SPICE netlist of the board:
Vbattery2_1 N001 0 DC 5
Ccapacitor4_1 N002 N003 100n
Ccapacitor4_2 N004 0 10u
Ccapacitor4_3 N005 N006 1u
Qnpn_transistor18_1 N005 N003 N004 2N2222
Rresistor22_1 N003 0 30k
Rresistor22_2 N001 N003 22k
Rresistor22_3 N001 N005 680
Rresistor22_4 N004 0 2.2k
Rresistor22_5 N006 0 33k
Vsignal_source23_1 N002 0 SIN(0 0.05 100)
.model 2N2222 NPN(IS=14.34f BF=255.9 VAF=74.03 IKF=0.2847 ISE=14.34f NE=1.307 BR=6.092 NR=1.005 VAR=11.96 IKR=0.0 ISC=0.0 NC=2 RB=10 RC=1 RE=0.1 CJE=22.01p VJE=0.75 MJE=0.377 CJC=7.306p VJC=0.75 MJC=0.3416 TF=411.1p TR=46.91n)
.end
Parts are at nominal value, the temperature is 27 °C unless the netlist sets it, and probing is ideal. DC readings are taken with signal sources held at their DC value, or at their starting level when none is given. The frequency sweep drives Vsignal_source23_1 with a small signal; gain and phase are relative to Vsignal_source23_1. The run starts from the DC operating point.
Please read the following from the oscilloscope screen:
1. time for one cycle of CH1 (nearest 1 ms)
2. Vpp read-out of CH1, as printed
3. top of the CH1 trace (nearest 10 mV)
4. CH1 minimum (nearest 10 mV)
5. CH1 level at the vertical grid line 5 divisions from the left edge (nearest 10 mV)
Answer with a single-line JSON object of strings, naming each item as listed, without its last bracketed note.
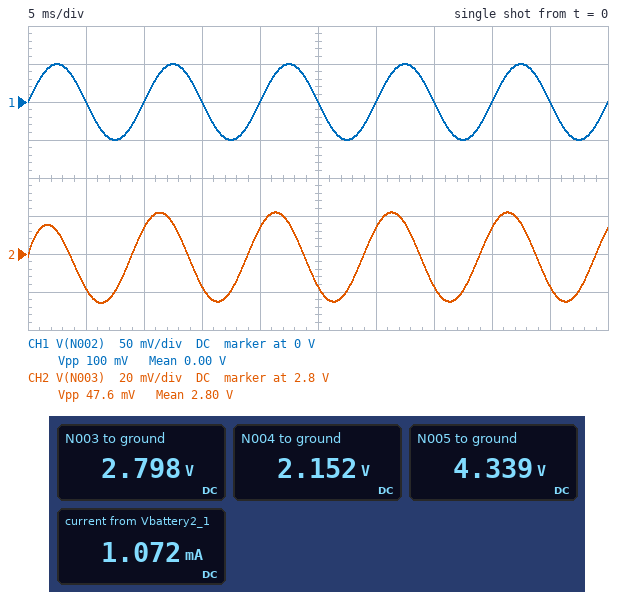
{"time for one cycle of CH1": "10 ms", "Vpp read-out of CH1, as printed": "100 mV", "top of the CH1 trace": "50 mV", "CH1 minimum": "-50 mV", "CH1 level at the vertical grid line 5 divisions from the left edge": "0 V"}
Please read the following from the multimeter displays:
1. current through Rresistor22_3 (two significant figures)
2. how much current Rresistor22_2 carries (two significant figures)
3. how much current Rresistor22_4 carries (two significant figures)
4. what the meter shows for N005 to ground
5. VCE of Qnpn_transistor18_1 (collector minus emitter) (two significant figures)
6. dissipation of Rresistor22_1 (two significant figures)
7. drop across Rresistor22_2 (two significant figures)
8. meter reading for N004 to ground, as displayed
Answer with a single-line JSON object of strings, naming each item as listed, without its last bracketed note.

{"current through Rresistor22_3": "970 µA", "how much current Rresistor22_2 carries": "100 µA", "how much current Rresistor22_4 carries": "980 µA", "what the meter shows for N005 to ground": "4.339 V", "VCE of Qnpn_transistor18_1 (collector minus emitter)": "2.2 V", "dissipation of Rresistor22_1": "260 µW", "drop across Rresistor22_2": "2.2 V", "meter reading for N004 to ground, as displayed": "2.152 V"}
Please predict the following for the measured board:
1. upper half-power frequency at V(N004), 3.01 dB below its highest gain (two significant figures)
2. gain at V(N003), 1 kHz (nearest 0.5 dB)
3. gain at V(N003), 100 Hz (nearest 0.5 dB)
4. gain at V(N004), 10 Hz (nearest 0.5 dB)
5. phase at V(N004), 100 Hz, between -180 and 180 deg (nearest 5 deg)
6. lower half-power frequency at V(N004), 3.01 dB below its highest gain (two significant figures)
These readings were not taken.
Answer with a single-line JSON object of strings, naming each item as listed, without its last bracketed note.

{"upper half-power frequency at V(N004), 3.01 dB below its highest gain": "1.2 kHz", "gain at V(N003), 1 kHz": "-2.0 dB", "gain at V(N003), 100 Hz": "-6.5 dB", "gain at V(N004), 10 Hz": "-22.5 dB", "phase at V(N004), 100 Hz, between -180 and 180 deg": "30 deg", "lower half-power frequency at V(N004), 3.01 dB below its highest gain": "67 Hz"}
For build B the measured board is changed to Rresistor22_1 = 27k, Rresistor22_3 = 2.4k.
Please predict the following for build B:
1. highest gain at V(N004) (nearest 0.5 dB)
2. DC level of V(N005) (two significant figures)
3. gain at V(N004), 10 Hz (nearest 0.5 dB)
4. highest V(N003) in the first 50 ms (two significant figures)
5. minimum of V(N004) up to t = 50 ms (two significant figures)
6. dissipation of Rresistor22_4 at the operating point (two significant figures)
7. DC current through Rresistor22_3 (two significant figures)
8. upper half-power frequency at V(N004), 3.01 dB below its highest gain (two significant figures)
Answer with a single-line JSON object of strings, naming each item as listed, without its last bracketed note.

{"highest gain at V(N004)": "-5.5 dB", "DC level of V(N005)": "2.8 V", "gain at V(N004), 10 Hz": "-23.0 dB", "highest V(N003) in the first 50 ms": "2.7 V", "minimum of V(N004) up to t = 50 ms": "2.0 V", "dissipation of Rresistor22_4 at the operating point": "1.9 mW", "DC current through Rresistor22_3": "920 µA", "upper half-power frequency at V(N004), 3.01 dB below its highest gain": "1.1 kHz"}
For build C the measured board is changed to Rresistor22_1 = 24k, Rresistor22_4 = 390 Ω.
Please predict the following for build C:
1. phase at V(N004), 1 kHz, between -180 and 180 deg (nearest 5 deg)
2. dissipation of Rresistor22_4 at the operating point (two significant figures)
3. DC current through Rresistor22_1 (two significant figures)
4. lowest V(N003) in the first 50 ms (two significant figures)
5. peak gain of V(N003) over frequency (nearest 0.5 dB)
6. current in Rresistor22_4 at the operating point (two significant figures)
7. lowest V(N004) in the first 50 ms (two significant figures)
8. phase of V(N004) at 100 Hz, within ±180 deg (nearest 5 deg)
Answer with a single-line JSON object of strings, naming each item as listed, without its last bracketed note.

{"phase at V(N004), 1 kHz, between -180 and 180 deg": "-10 deg", "dissipation of Rresistor22_4 at the operating point": "6.7 mW", "DC current through Rresistor22_1": "96 µA", "lowest V(N003) in the first 50 ms": "2.3 V", "peak gain of V(N003) over frequency": "0 dB", "current in Rresistor22_4 at the operating point": "4.2 mA", "lowest V(N004) in the first 50 ms": "1.6 V", "phase of V(N004) at 100 Hz, within ±180 deg": "45 deg"}
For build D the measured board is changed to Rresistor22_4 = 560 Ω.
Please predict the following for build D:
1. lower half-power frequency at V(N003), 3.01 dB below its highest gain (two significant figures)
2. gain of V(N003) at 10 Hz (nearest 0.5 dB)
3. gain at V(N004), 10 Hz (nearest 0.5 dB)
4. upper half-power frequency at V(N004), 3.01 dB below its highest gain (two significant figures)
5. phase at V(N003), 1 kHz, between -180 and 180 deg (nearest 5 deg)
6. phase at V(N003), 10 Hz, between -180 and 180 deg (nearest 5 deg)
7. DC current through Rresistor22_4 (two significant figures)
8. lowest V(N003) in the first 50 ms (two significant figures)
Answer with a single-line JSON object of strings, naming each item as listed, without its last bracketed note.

{"lower half-power frequency at V(N003), 3.01 dB below its highest gain": "1.6 kHz", "gain of V(N003) at 10 Hz": "-23.0 dB", "gain at V(N004), 10 Hz": "-23.5 dB", "upper half-power frequency at V(N004), 3.01 dB below its highest gain": "3.4 kHz", "phase at V(N003), 1 kHz, between -180 and 180 deg": "15 deg", "phase at V(N003), 10 Hz, between -180 and 180 deg": "85 deg", "DC current through Rresistor22_4": "3.4 mA", "lowest V(N003) in the first 50 ms": "2.6 V"}
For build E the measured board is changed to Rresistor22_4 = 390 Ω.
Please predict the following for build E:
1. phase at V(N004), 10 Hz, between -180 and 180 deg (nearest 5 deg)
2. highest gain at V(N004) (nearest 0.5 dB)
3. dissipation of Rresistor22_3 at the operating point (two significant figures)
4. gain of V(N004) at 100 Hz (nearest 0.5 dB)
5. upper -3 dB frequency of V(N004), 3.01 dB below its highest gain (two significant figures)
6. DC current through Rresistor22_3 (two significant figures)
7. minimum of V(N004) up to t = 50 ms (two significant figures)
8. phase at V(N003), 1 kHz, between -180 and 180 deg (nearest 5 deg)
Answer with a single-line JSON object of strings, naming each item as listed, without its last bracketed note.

{"phase at V(N004), 10 Hz, between -180 and 180 deg": "80 deg", "highest gain at V(N004)": "-21.0 dB", "dissipation of Rresistor22_3 at the operating point": "14 mW", "gain of V(N004) at 100 Hz": "-22.5 dB", "upper -3 dB frequency of V(N004), 3.01 dB below its highest gain": "17 kHz", "DC current through Rresistor22_3": "4.5 mA", "minimum of V(N004) up to t = 50 ms": "1.8 V", "phase at V(N003), 1 kHz, between -180 and 180 deg": "30 deg"}
